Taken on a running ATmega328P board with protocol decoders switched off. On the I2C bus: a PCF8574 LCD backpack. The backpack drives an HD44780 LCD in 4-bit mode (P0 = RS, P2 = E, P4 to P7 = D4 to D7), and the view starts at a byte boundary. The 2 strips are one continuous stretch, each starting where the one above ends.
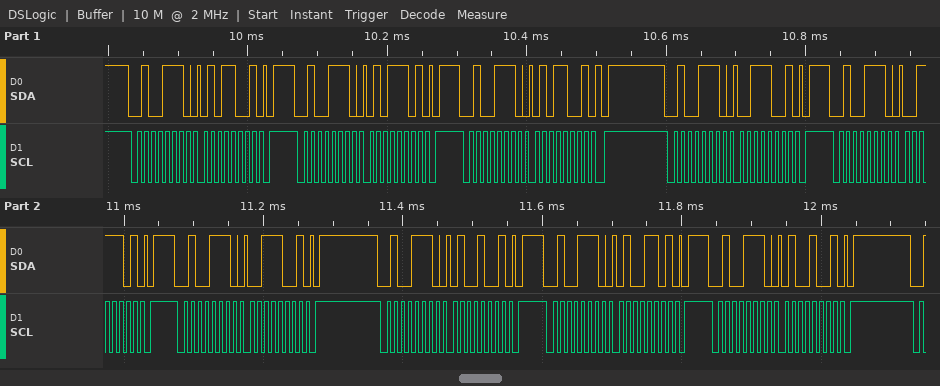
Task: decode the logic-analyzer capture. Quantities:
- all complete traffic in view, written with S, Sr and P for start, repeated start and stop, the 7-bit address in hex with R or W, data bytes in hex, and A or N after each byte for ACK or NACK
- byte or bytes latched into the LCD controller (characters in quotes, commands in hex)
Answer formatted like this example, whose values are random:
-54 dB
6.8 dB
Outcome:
S 27W A 59 A P S 27W A 5D A P S 27W A 59 A P S 27W A 39 A P S 27W A 3D A P S 27W A 39 A P S 27W A 49 A P S 27W A 4D A P S 27W A 49 A P
'S'
